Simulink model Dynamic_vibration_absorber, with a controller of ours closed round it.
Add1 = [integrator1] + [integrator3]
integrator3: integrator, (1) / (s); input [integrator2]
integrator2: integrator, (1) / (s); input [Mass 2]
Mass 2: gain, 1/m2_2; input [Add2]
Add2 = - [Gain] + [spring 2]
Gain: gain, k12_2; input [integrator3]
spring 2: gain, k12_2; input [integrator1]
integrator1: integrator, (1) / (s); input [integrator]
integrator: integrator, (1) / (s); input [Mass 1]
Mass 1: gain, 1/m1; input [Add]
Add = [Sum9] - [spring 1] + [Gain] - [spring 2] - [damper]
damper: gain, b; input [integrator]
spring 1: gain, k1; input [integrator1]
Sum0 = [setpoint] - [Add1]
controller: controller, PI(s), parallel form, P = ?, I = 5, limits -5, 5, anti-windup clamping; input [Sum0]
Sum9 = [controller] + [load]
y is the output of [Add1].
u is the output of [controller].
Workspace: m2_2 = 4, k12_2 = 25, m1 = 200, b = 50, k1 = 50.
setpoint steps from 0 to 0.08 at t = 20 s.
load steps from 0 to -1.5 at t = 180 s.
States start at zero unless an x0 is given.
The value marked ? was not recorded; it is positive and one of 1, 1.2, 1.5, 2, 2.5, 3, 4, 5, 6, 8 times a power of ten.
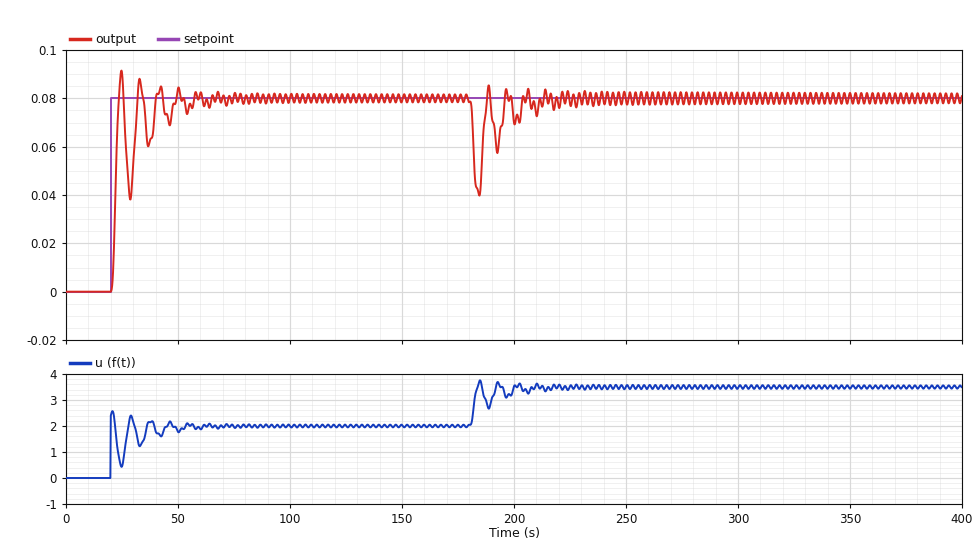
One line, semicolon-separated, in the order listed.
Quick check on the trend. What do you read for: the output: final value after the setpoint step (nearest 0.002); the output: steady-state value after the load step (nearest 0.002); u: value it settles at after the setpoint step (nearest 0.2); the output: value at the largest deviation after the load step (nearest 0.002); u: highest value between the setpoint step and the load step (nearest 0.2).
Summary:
0.080; 0.080; 2.0; 0.040; 2.6
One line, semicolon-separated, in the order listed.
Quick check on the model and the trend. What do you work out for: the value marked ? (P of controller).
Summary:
30
